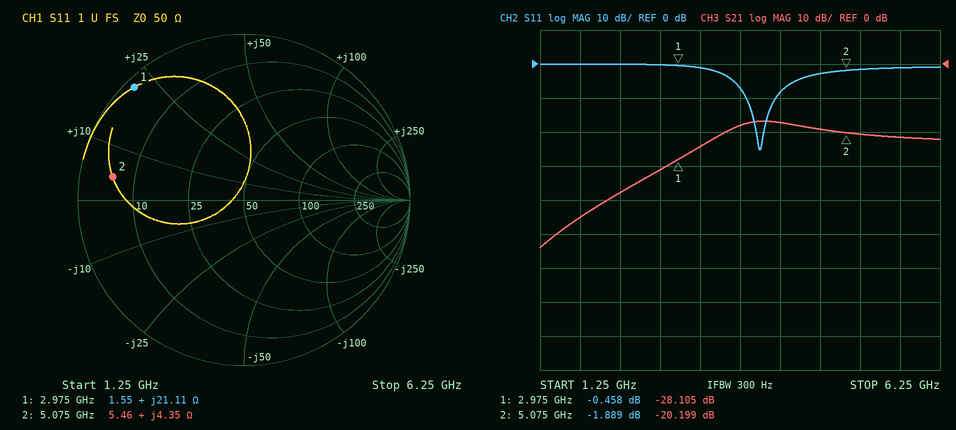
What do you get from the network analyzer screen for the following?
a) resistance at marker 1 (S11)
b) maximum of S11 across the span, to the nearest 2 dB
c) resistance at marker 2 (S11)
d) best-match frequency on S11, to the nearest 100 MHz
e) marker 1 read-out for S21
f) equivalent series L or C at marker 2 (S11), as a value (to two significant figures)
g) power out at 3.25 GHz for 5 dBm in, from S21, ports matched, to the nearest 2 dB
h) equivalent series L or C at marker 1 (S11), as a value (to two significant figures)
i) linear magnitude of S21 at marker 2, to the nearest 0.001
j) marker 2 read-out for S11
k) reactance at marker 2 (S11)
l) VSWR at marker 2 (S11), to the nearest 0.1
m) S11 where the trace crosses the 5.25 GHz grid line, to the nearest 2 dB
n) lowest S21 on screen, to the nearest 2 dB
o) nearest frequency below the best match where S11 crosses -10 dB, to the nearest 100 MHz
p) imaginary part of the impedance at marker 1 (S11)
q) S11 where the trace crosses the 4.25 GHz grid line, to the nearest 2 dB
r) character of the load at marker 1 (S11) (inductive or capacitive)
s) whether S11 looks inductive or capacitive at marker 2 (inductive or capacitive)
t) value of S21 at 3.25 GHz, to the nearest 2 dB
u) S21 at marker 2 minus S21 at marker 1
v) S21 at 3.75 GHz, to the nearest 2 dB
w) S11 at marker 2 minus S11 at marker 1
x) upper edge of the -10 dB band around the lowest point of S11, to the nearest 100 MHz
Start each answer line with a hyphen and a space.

- 1.55 Ω
- 0 dB
- 5.46 Ω
- 4.0 GHz
- -28.105 dB
- 140 pH
- -20 dBm
- 1.1 nH
- 0.098
- -1.889 dB
- +4.35 Ω
- 9.2
- -2 dB
- -54 dB
- 3.8 GHz
- +21.11 Ω
- -8 dB
- inductive
- inductive
- -24 dB
- 7.906 dB
- -18 dB
- -1.431 dB
- 4.2 GHz
